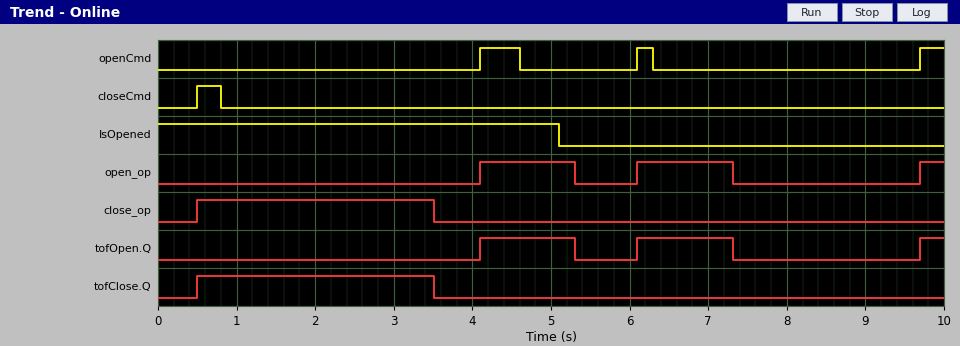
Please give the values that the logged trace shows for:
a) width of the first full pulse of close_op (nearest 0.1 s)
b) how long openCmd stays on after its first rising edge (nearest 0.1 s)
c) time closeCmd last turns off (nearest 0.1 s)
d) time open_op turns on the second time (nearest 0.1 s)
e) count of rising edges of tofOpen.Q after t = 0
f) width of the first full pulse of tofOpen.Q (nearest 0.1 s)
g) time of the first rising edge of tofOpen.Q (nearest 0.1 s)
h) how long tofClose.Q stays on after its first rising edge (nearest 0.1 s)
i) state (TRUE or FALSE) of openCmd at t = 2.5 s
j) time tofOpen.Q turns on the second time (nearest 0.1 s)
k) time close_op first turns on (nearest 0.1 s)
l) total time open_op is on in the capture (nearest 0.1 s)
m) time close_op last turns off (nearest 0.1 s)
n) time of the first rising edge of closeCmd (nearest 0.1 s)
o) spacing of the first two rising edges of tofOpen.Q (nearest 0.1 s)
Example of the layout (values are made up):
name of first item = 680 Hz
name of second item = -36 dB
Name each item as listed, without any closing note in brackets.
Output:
width of the first full pulse of close_op = 3.0 s
how long openCmd stays on after its first rising edge = 0.5 s
time closeCmd last turns off = 0.8 s
time open_op turns on the second time = 6.1 s
count of rising edges of tofOpen.Q after t = 0 = 3
width of the first full pulse of tofOpen.Q = 1.2 s
time of the first rising edge of tofOpen.Q = 4.1 s
how long tofClose.Q stays on after its first rising edge = 3.0 s
state (TRUE or FALSE) of openCmd at t = 2.5 s = FALSE
time tofOpen.Q turns on the second time = 6.1 s
time close_op first turns on = 0.5 s
total time open_op is on in the capture = 2.7 s
time close_op last turns off = 3.5 s
time of the first rising edge of closeCmd = 0.5 s
spacing of the first two rising edges of tofOpen.Q = 2.0 s
